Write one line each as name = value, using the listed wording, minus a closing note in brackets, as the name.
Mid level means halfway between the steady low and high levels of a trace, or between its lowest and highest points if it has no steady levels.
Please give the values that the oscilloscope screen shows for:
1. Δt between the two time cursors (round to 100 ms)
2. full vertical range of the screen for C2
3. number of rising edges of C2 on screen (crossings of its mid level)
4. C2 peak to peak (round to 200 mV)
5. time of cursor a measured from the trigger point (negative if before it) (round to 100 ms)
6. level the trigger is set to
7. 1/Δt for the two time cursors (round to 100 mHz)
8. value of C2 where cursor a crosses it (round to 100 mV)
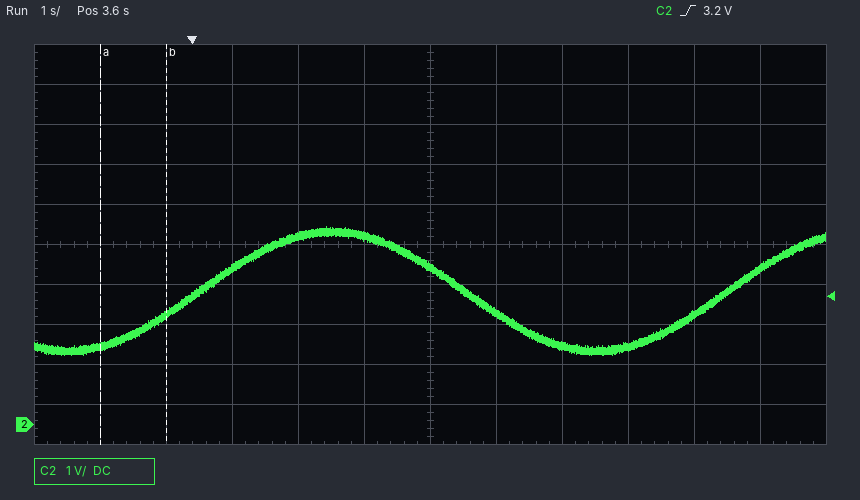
Δt between the two time cursors = 1.0 s
full vertical range of the screen for C2 = 10 V
number of rising edges of C2 on screen = 2
C2 peak to peak = 3.2 V
time of cursor a measured from the trigger point (negative if before it) = -1.4 s
level the trigger is set to = 3.2 V
1/Δt for the two time cursors = 1.0 Hz
value of C2 where cursor a crosses it = 2.0 V
